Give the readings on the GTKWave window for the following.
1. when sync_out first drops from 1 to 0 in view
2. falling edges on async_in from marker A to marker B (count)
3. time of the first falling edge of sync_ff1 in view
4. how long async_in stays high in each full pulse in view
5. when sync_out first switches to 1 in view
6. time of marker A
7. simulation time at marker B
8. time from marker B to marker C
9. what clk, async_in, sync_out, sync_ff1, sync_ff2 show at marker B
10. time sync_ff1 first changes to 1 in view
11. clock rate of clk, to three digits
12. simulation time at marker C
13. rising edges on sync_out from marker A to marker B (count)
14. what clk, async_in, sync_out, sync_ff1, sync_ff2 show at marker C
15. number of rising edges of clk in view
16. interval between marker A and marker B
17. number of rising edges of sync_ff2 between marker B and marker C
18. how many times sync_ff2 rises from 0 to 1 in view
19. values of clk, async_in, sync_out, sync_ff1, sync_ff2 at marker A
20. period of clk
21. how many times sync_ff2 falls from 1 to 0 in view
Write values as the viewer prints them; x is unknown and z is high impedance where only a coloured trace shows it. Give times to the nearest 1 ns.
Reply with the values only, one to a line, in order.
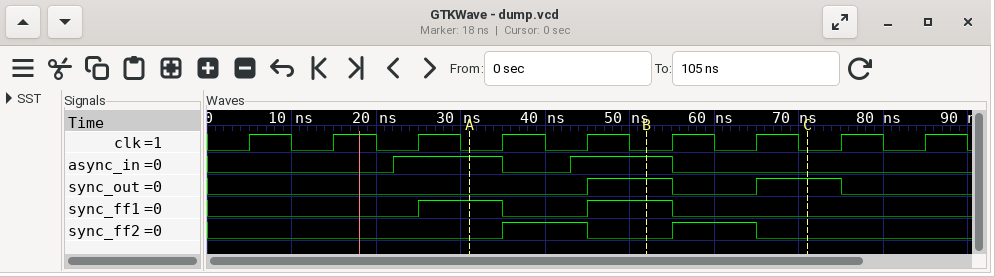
55 ns
1
35 ns
13 ns, 12 ns
45 ns
31 ns
52 ns
19 ns
clk=0, async_in=1, sync_out=1, sync_ff1=1, sync_ff2=0
25 ns
100 MHz
71 ns
1
clk=0, async_in=0, sync_out=1, sync_ff1=0, sync_ff2=0
9
21 ns
1
2
clk=0, async_in=1, sync_out=0, sync_ff1=1, sync_ff2=0
10 ns
2
